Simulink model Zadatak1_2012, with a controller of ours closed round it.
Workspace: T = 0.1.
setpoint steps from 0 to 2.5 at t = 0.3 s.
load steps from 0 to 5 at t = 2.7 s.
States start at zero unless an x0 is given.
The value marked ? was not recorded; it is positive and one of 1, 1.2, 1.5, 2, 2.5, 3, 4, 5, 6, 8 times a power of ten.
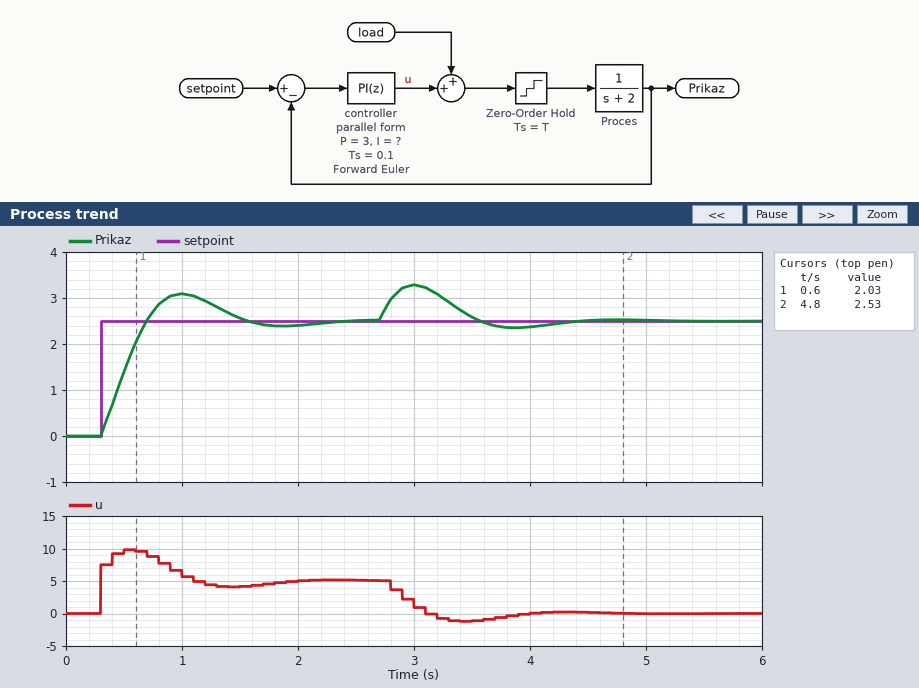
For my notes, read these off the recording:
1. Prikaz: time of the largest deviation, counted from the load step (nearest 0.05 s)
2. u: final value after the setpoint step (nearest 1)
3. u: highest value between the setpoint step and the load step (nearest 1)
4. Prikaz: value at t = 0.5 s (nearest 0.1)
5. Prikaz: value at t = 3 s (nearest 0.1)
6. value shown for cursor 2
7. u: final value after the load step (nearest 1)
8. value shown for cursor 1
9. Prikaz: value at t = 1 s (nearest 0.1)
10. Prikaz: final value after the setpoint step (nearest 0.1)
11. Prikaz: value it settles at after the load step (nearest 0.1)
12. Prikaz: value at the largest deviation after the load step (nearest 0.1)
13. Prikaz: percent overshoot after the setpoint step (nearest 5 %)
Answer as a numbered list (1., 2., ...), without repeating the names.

1. 0.30 s
2. 5
3. 10
4. 1.4
5. 3.3
6. 2.53
7. 0
8. 2.03
9. 3.1
10. 2.5
11. 2.5
12. 3.3
13. 25 %
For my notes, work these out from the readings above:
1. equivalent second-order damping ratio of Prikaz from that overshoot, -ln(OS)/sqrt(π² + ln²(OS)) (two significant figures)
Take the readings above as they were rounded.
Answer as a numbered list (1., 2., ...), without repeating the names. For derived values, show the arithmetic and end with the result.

1. ln(0.25) = -1.386; 1.386 / sqrt(9.870 + 1.922) = 0.40
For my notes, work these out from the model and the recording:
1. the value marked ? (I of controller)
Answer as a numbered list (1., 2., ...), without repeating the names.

1. 15
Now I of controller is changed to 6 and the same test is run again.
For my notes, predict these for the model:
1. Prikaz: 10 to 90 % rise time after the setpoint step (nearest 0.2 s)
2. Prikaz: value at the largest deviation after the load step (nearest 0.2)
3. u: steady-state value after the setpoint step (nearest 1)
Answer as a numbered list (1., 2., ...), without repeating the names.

1. 0.6 s
2. 3.4
3. 5
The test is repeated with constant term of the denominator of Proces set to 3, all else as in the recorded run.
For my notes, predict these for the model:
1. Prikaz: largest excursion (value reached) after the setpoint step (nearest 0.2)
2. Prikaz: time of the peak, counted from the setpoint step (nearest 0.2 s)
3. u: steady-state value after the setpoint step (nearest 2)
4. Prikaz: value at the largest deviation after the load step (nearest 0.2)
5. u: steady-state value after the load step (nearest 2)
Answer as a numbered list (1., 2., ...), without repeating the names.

1. 2.8
2. 0.8 s
3. 8
4. 3.2
5. 2
